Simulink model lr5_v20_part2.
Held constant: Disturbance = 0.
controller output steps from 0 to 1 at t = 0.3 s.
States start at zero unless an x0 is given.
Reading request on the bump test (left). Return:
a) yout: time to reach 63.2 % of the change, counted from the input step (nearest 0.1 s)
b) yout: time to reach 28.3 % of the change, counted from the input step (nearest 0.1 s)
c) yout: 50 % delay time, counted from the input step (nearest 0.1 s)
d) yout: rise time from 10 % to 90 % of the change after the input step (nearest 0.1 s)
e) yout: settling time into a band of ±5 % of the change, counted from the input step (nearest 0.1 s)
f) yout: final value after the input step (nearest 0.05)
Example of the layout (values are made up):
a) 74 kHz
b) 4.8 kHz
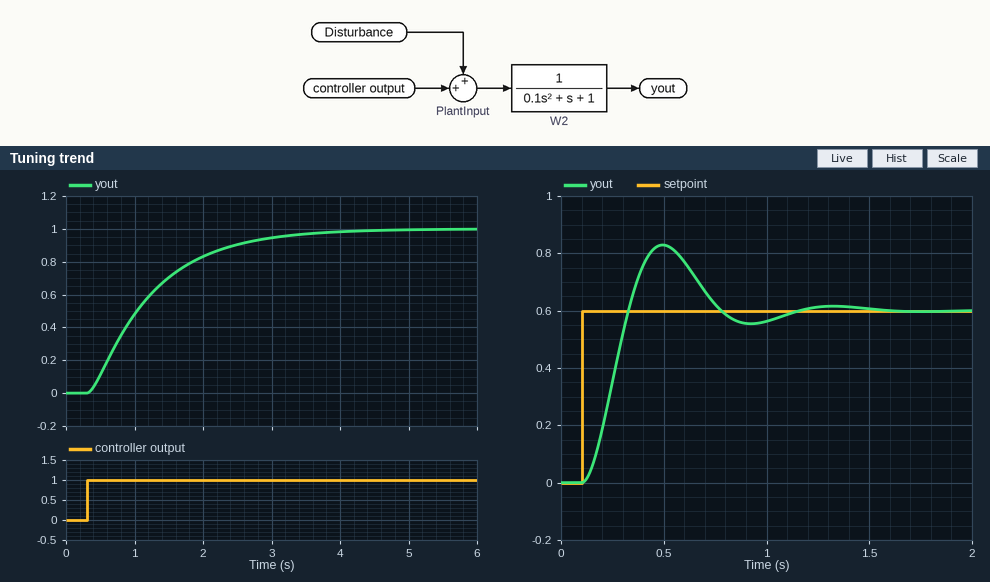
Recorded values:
a) 1.0 s
b) 0.4 s
c) 0.7 s
d) 2.0 s
e) 2.8 s
f) 1.00
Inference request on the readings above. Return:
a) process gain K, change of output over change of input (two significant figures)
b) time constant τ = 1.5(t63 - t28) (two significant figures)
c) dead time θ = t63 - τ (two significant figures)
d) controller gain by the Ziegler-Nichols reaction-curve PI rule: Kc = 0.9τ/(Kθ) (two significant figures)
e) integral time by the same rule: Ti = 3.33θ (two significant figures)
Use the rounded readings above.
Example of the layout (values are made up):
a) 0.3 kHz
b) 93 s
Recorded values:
a) 1.0
b) 0.90 s
c) 0.10 s
d) 8.1
e) 0.33 s
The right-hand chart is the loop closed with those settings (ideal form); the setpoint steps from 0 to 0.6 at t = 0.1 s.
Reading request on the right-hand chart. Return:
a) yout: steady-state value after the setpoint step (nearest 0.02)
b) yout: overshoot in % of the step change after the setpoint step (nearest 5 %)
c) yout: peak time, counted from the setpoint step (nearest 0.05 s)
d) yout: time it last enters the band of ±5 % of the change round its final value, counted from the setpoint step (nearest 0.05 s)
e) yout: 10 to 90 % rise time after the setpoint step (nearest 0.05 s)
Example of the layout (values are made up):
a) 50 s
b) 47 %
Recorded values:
a) 0.60
b) 40 %
c) 0.40 s
d) 0.95 s
e) 0.15 s
